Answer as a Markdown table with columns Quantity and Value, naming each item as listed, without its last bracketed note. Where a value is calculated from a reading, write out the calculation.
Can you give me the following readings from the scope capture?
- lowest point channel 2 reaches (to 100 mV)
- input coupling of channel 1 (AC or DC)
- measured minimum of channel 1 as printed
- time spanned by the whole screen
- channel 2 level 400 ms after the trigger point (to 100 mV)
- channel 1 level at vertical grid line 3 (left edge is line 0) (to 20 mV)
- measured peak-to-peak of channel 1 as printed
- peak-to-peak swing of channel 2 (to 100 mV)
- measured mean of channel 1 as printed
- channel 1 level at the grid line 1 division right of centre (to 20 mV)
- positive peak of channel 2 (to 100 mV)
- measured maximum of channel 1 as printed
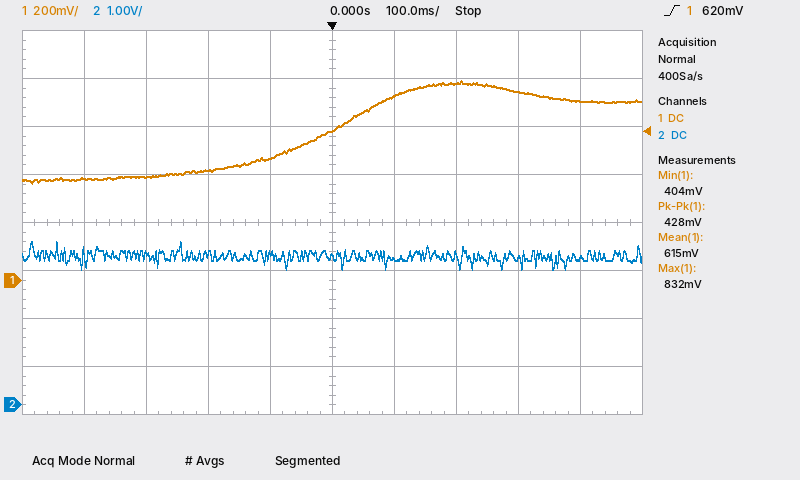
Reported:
| Quantity | Value |
|---|---|
| lowest point channel 2 reaches | 2.8 V |
| input coupling of channel 1 | DC |
| measured minimum of channel 1 as printed | 404 mV |
| time spanned by the whole screen | 1 s |
| channel 2 level 400 ms after the trigger point | 3.1 V |
| channel 1 level at vertical grid line 3 (left edge is line 0) | 460 mV |
| measured peak-to-peak of channel 1 as printed | 428 mV |
| peak-to-peak swing of channel 2 | 3.4 V − (2.8 V) = 600 mV |
| measured mean of channel 1 as printed | 615 mV |
| channel 1 level at the grid line 1 division right of centre | 760 mV |
| positive peak of channel 2 | 3.4 V |
| measured maximum of channel 1 as printed | 832 mV |
